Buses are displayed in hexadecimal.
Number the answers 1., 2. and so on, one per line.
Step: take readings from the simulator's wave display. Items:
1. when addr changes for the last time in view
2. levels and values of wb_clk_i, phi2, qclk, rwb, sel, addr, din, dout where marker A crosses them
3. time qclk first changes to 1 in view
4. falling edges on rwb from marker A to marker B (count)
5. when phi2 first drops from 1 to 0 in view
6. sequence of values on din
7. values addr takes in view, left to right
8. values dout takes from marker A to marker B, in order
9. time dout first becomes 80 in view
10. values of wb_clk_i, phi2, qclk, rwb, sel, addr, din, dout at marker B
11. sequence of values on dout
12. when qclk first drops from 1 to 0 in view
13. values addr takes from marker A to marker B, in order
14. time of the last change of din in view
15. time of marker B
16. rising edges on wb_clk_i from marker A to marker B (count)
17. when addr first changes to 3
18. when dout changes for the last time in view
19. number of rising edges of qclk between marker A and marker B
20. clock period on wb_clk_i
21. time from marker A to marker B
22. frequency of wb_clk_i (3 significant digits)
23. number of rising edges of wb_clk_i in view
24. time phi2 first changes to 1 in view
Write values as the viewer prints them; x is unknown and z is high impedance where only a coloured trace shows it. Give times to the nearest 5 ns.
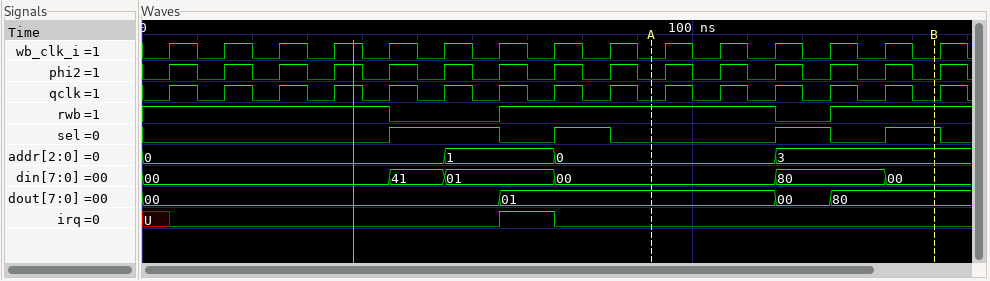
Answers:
1. 115 ns
2. wb_clk_i=0, phi2=0, qclk=0, rwb=1, sel=0, addr=0, din=00, dout=01
3. 5 ns
4. 1
5. 10 ns
6. 00, 41, 01, 00, 80, 00
7. 0, 1, 0, 3
8. 01, 00, 80
9. 125 ns
10. wb_clk_i=0, phi2=0, qclk=0, rwb=1, sel=1, addr=3, din=00, dout=80
11. 00, 01, 00, 80
12. 10 ns
13. 0, 3
14. 135 ns
15. 145 ns
16. 5
17. 115 ns
18. 125 ns
19. 5
20. 10 ns
21. 50 ns
22. 100 MHz
23. 15
24. 5 ns
